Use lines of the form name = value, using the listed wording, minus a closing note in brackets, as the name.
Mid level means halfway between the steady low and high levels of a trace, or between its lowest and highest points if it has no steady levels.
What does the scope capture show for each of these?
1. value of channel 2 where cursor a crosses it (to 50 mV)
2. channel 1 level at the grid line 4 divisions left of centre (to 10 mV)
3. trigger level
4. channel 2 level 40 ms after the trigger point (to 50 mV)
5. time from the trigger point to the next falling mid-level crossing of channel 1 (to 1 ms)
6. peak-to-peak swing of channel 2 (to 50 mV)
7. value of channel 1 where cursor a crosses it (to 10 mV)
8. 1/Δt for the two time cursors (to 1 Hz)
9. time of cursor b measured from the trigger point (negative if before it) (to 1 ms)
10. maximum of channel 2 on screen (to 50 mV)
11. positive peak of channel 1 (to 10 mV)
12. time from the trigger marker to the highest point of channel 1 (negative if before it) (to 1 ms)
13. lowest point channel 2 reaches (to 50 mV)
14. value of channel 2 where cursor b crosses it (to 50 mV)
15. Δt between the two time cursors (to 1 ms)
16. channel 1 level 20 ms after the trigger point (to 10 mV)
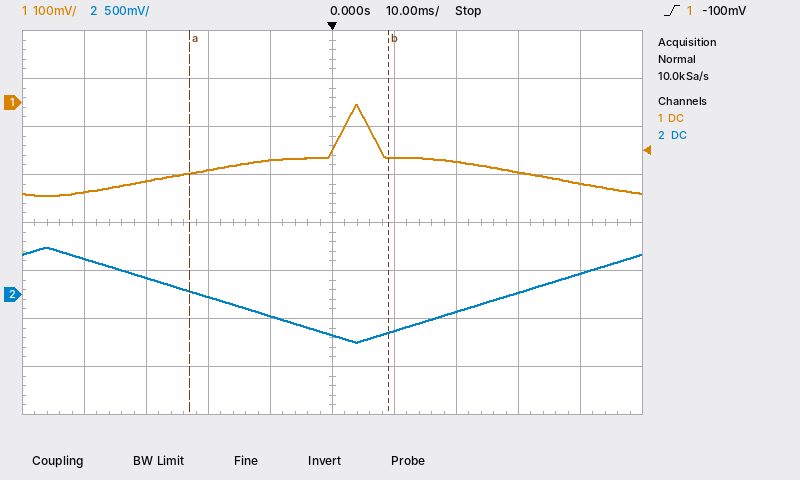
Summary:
value of channel 2 where cursor a crosses it = 50 mV
channel 1 level at the grid line 4 divisions left of centre = -190 mV
trigger level = -100 mV
channel 2 level 40 ms after the trigger point = 200 mV
time from the trigger point to the next falling mid-level crossing of channel 1 = 8 ms
peak-to-peak swing of channel 2 = 1.00 V
value of channel 1 where cursor a crosses it = -150 mV
1/Δt for the two time cursors = 31 Hz
time of cursor b measured from the trigger point (negative if before it) = +9 ms
maximum of channel 2 on screen = 500 mV
positive peak of channel 1 = 0 mV
time from the trigger marker to the highest point of channel 1 (negative if before it) = +4 ms
lowest point channel 2 reaches = -500 mV
value of channel 2 where cursor b crosses it = -400 mV
Δt between the two time cursors = 32 ms
channel 1 level 20 ms after the trigger point = -120 mV
